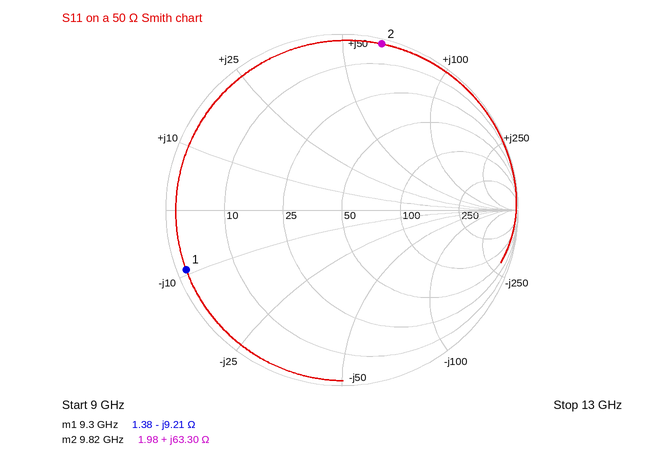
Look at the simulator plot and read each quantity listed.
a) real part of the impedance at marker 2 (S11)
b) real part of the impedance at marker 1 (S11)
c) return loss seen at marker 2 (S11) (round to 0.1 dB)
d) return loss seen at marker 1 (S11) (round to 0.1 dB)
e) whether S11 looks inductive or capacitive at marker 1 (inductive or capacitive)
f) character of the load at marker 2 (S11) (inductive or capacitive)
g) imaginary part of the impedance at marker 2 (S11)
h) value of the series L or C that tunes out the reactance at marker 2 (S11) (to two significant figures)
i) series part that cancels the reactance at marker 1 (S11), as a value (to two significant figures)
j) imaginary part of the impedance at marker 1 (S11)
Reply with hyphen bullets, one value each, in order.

- 1.98 Ω
- 1.38 Ω
- 0.3 dB
- 0.5 dB
- capacitive
- inductive
- +63.30 Ω
- 260 fF
- 160 pH
- -9.21 Ω
